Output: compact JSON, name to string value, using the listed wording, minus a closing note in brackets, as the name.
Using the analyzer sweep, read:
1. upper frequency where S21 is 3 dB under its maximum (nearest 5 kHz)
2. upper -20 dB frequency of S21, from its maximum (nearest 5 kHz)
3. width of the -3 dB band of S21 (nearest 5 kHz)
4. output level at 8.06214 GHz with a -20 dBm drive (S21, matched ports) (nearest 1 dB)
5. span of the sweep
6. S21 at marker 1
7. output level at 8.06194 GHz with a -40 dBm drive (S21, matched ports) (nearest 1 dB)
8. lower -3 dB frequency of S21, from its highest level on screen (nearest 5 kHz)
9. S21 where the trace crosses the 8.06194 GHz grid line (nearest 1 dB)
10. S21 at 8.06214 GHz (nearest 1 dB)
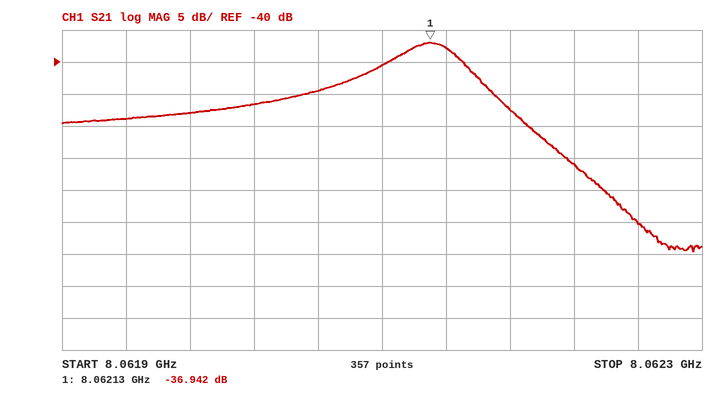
{"upper frequency where S21 is 3 dB under its maximum": "8.062150 GHz", "upper -20 dB frequency of S21, from its maximum": "8.062225 GHz", "width of the -3 dB band of S21": "45 kHz", "output level at 8.06214 GHz with a -20 dBm drive (S21, matched ports)": "-58 dBm", "span of the sweep": "400 kHz", "S21 at marker 1": "-36.942 dB", "output level at 8.06194 GHz with a -40 dBm drive (S21, matched ports)": "-89 dBm", "lower -3 dB frequency of S21, from its highest level on screen": "8.062105 GHz", "S21 where the trace crosses the 8.06194 GHz grid line": "-49 dB", "S21 at 8.06214 GHz": "-38 dB"}
